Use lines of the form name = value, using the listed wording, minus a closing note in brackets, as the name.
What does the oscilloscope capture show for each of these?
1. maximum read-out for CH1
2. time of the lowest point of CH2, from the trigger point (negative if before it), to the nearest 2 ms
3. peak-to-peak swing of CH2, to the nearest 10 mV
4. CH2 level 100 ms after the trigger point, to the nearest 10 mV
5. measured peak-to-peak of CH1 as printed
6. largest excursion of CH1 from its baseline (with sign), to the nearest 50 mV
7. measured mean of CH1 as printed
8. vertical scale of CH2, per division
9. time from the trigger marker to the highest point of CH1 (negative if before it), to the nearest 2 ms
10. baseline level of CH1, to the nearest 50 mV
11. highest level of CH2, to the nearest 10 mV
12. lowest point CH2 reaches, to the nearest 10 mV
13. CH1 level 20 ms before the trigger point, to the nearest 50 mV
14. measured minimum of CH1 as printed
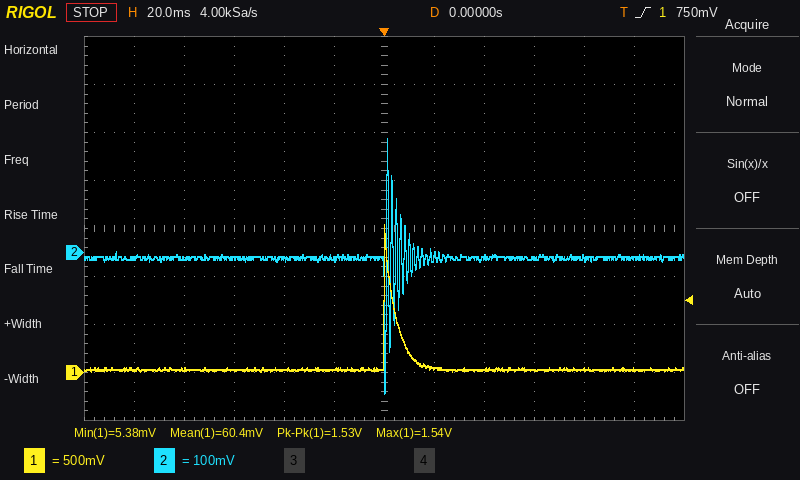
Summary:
maximum read-out for CH1 = 1.54 V
time of the lowest point of CH2, from the trigger point (negative if before it), to the nearest 2 ms = 0 ms
peak-to-peak swing of CH2, to the nearest 10 mV = 530 mV
CH2 level 100 ms after the trigger point, to the nearest 10 mV = -10 mV
measured peak-to-peak of CH1 as printed = 1.53 V
largest excursion of CH1 from its baseline (with sign), to the nearest 50 mV = +1.50 V
measured mean of CH1 as printed = 60.4 mV
vertical scale of CH2, per division = 100 mV
time from the trigger marker to the highest point of CH1 (negative if before it), to the nearest 2 ms = 0 ms
baseline level of CH1, to the nearest 50 mV = 50 mV
highest level of CH2, to the nearest 10 mV = 240 mV
lowest point CH2 reaches, to the nearest 10 mV = -290 mV
CH1 level 20 ms before the trigger point, to the nearest 50 mV = 50 mV
measured minimum of CH1 as printed = 5.38 mV
